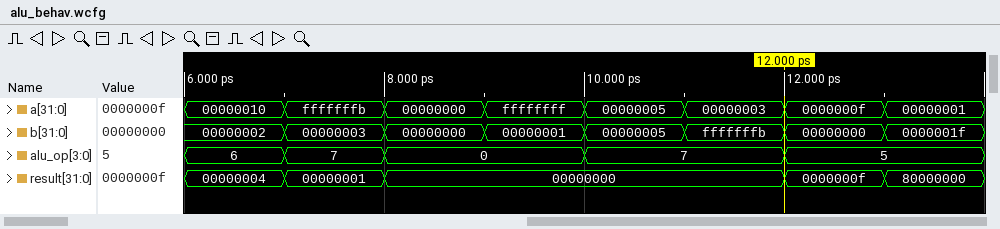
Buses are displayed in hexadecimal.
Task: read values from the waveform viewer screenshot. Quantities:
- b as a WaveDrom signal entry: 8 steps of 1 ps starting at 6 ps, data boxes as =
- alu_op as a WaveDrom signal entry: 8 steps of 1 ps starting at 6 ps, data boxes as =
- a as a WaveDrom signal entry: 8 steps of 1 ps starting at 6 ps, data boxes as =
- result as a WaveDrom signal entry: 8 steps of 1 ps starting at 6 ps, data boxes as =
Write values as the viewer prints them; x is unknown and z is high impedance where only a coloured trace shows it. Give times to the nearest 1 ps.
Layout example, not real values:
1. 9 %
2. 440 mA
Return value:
1. {name: 'b', wave: '========', data: '00000002 00000003 00000000 00000001 00000005 fffffffb 00000000 0000001f'}
2. {name: 'alu_op', wave: '===.=.=.', data: '6 7 0 7 5'}
3. {name: 'a', wave: '========', data: '00000010 fffffffb 00000000 ffffffff 00000005 00000003 0000000f 00000001'}
4. {name: 'result', wave: '===...==', data: '00000004 00000001 00000000 0000000f 80000000'}
